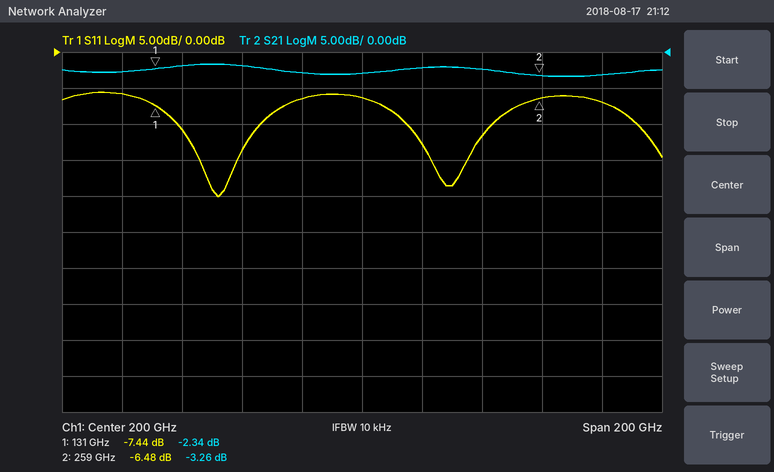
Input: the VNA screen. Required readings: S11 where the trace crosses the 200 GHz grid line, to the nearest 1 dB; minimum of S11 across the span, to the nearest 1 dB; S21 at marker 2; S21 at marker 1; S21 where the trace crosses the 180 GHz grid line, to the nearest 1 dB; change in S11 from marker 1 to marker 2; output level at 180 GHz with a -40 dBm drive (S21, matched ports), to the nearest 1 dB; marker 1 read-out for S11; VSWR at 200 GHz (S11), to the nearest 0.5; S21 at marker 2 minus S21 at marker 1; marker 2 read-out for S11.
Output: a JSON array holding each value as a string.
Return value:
["-6 dB", "-20 dB", "-3.26 dB", "-2.34 dB", "-3 dB", "0.96 dB", "-43 dBm", "-7.44 dB", "3.0", "-0.92 dB", "-6.48 dB"]
